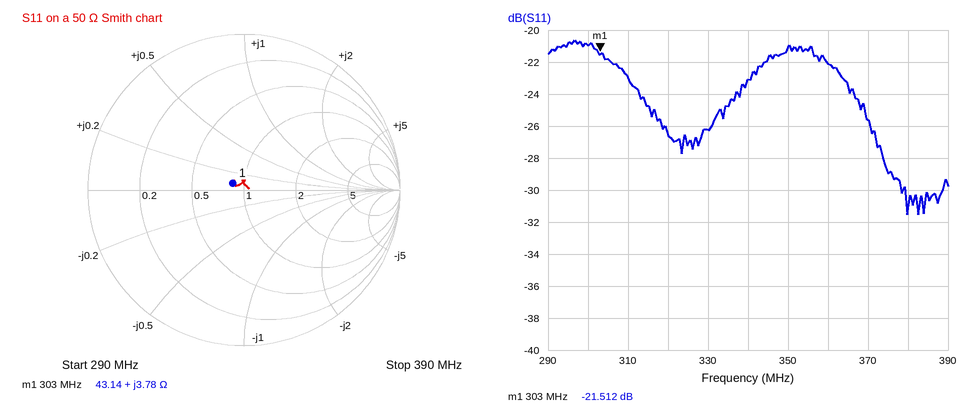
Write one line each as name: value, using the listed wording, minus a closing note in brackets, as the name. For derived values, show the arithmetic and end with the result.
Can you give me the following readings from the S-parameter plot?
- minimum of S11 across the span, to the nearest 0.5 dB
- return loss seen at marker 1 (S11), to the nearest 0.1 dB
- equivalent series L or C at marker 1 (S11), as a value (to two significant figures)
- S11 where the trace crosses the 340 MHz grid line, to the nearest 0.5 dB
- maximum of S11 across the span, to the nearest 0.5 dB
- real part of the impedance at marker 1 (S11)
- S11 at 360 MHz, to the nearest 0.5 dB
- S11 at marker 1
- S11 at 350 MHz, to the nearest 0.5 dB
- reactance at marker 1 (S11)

minimum of S11 across the span, to the nearest 0.5 dB: -31.5 dB
return loss seen at marker 1 (S11), to the nearest 0.1 dB: 21.5 dB
equivalent series L or C at marker 1 (S11), as a value: L = 3.78 Ω/(2π × 303 MHz) ≈ 2.0 nH
S11 where the trace crosses the 340 MHz grid line, to the nearest 0.5 dB: -23.0 dB
maximum of S11 across the span, to the nearest 0.5 dB: -20.5 dB
real part of the impedance at marker 1: 43.14 Ω
S11 at 360 MHz, to the nearest 0.5 dB: -22.0 dB
S11 at marker 1: -21.512 dB
S11 at 350 MHz, to the nearest 0.5 dB: -21.0 dB
reactance at marker 1: +3.78 Ω
